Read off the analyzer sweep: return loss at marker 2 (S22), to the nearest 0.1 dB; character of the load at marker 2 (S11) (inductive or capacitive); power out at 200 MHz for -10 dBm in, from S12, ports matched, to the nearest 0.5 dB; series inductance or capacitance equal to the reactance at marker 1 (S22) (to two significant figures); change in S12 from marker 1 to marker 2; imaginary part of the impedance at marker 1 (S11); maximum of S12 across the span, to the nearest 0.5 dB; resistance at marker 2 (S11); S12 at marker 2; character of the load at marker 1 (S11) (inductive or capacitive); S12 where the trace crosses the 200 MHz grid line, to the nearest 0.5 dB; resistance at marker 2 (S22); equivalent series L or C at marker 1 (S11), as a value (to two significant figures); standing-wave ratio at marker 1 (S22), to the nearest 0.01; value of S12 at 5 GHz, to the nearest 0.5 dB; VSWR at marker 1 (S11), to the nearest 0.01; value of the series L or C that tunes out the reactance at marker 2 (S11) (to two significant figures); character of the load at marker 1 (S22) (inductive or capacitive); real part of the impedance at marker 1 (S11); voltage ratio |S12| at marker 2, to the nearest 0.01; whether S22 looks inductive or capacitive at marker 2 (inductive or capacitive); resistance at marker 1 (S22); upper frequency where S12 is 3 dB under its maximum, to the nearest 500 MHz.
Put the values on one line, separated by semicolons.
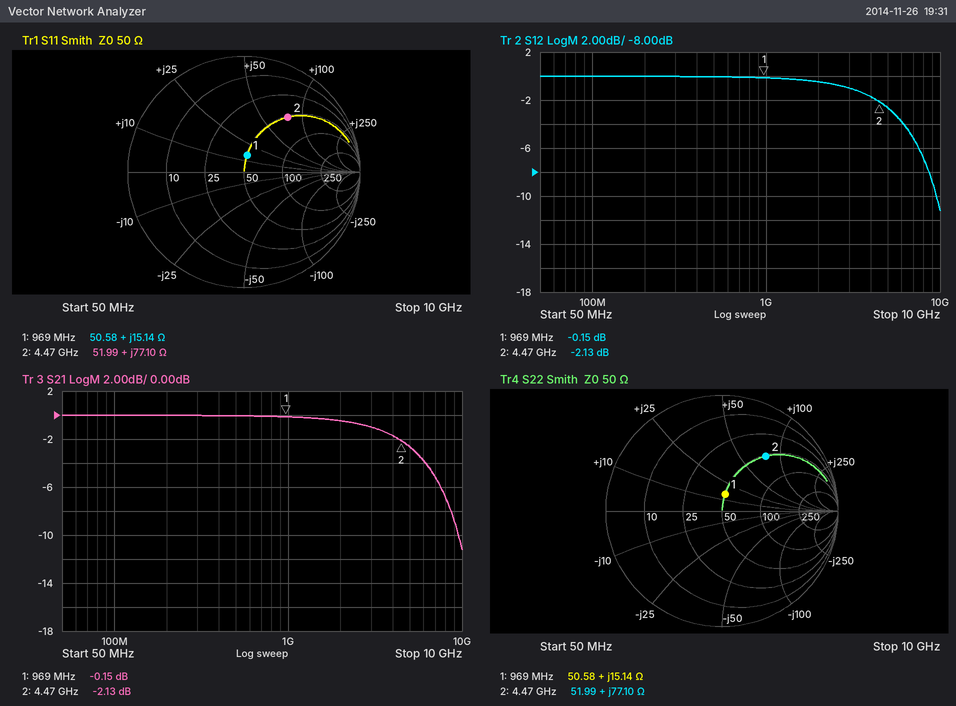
4.4 dB; inductive; -10.0 dBm; 2.5 nH; -1.98 dB; +15.14 Ω; 0.0 dB; 51.99 Ω; -2.13 dB; inductive; 0.0 dB; 51.99 Ω; 2.5 nH; 1.35; -2.5 dB; 1.35; 460 fF; inductive; 50.58 Ω; 0.78; inductive; 50.58 Ω; 5.5 GHz
